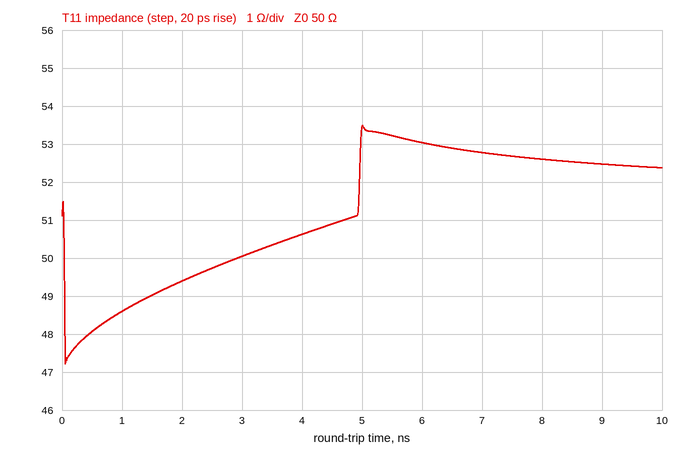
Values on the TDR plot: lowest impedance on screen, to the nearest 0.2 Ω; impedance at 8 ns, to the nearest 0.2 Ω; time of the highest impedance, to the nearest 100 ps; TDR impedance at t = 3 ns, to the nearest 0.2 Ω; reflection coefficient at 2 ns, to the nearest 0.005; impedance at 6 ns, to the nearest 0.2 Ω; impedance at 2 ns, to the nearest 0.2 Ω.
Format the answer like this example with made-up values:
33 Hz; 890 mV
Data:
47.2 Ω; 52.6 Ω; 5.0 ns; 50.0 Ω; -0.005; 53.0 Ω; 49.4 Ω
